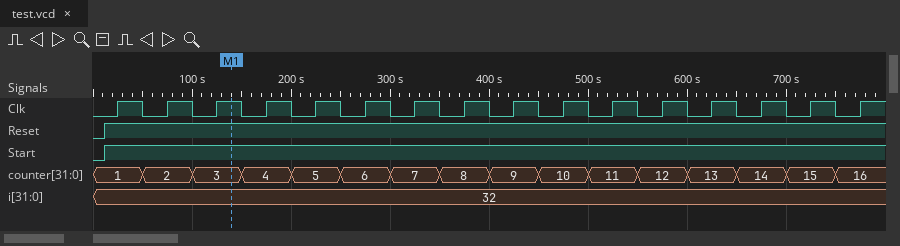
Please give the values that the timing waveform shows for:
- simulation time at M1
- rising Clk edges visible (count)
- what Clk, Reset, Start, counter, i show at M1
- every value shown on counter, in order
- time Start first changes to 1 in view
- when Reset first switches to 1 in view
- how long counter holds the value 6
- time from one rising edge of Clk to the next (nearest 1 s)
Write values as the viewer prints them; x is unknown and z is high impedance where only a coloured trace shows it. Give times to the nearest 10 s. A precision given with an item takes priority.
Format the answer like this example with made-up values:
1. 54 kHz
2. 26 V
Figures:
1. 140 s
2. 16
3. Clk=1, Reset=1, Start=1, counter=3, i=32
4. 1, 2, 3, 4, 5, 6, 7, 8, 9, 10, 11, 12, 13, 14, 15, 16
5. 10 s
6. 10 s
7. 50 s
8. 50 s
